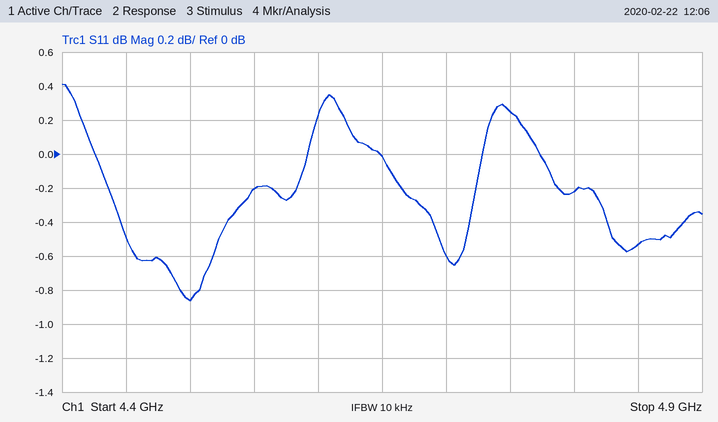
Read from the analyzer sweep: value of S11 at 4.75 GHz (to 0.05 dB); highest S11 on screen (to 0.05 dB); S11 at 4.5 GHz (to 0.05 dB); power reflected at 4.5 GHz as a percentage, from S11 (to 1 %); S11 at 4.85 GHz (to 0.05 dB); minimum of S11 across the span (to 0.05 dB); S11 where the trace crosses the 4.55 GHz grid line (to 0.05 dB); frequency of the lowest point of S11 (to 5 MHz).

0.25 dB
0.40 dB
-0.85 dB
82 %
-0.55 dB
-0.85 dB
-0.20 dB
4.500 GHz
